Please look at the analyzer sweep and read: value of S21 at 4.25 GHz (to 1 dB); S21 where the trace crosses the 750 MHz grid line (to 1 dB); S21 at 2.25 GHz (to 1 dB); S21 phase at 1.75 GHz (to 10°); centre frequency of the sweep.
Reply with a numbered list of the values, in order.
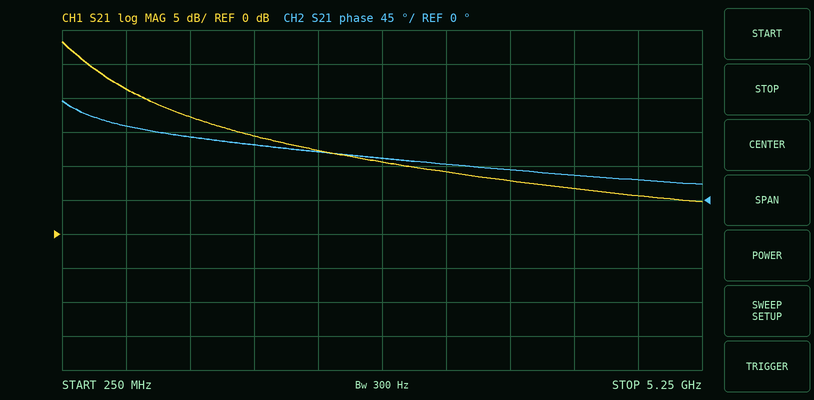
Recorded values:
1. 7 dB
2. 21 dB
3. 12 dB
4. 70°
5. 2.75 GHz
